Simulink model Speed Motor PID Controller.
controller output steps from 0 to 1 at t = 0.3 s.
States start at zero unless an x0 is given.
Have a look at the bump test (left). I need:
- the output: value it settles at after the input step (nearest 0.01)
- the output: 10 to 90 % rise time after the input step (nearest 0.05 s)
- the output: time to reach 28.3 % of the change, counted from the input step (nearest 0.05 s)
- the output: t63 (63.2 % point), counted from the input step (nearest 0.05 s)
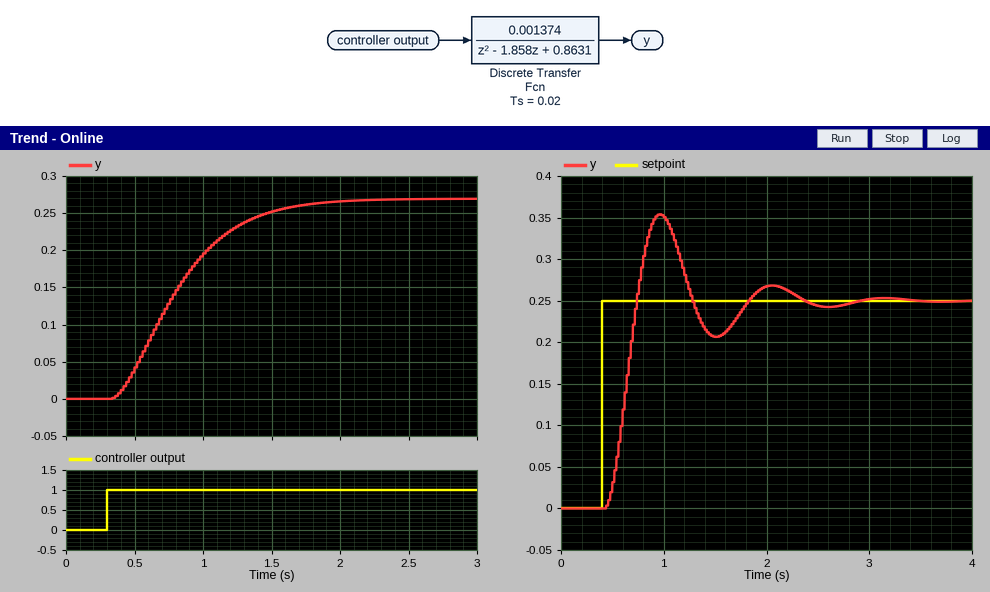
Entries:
0.27
0.90 s
0.30 s
0.60 s
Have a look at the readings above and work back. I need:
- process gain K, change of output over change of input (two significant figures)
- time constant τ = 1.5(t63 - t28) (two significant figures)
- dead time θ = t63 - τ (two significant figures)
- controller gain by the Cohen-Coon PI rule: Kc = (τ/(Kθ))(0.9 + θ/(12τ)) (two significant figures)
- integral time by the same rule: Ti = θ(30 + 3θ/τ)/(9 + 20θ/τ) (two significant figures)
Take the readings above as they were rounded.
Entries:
0.27
0.45 s
0.15 s
10
0.30 s
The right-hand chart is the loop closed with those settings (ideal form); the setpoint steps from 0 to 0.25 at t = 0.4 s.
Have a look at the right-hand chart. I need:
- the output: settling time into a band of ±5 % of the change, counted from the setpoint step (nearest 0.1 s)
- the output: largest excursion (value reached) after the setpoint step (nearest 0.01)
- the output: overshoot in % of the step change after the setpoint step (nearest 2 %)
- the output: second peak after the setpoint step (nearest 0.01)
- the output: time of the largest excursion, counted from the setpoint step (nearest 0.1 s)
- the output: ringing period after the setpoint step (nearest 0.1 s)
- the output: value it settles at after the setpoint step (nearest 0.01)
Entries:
1.8 s
0.35
42 %
0.27
0.6 s
1.1 s
0.25
